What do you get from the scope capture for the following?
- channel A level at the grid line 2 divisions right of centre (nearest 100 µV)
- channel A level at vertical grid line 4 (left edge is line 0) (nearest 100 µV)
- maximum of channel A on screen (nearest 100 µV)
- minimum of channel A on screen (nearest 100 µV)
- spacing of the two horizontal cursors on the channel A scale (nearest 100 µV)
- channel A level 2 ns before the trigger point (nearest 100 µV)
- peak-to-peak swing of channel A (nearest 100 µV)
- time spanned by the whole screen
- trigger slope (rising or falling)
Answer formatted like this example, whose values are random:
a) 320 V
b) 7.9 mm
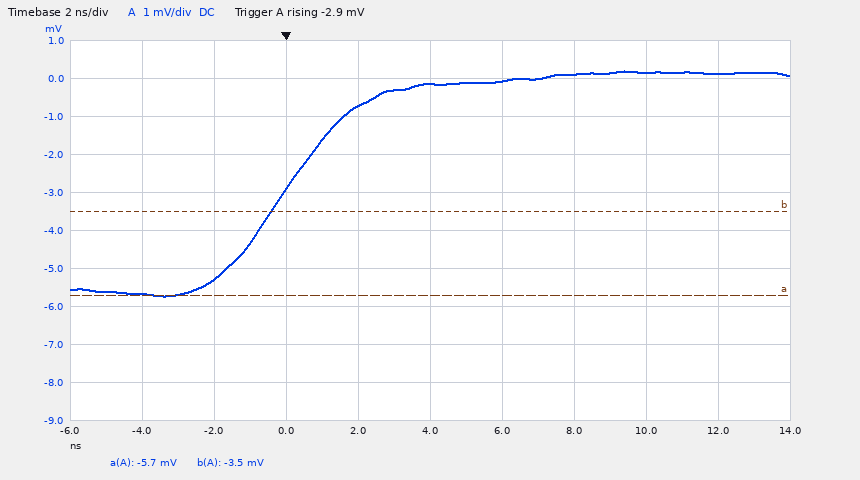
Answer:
a) 100 µV
b) -700 µV
c) 200 µV
d) -5.7 mV
e) 2.2 mV
f) -5.3 mV
g) 5.9 mV
h) 20 ns
i) rising
